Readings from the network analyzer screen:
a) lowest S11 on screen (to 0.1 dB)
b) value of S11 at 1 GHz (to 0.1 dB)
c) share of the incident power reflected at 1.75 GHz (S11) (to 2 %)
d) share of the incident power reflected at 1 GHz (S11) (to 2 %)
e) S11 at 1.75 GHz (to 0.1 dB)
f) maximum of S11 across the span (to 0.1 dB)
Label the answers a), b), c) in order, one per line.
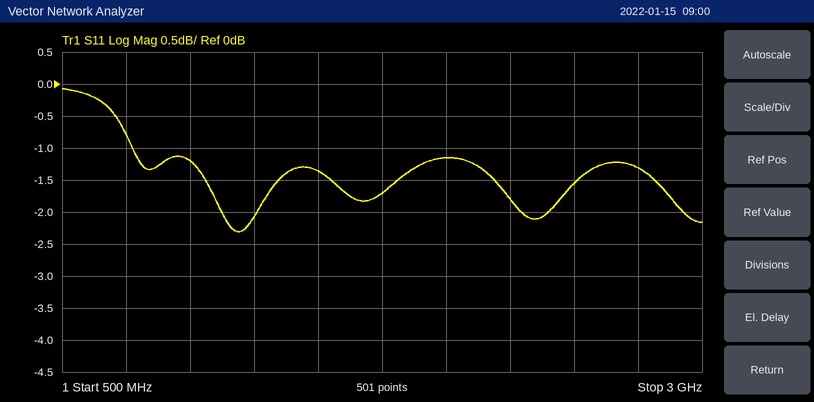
a) -2.3 dB
b) -1.2 dB
c) 68 %
d) 76 %
e) -1.7 dB
f) -0.1 dB
